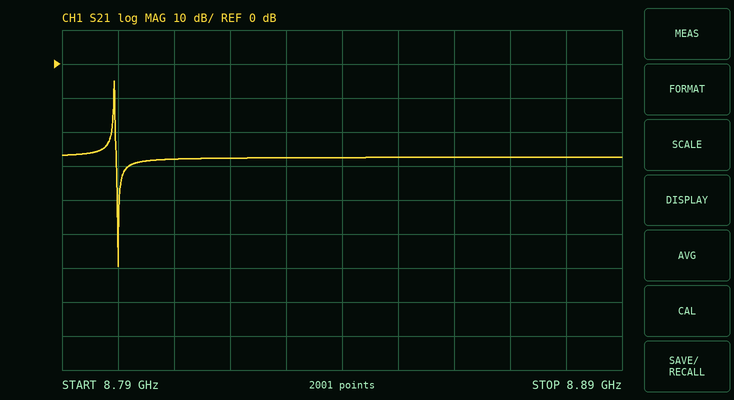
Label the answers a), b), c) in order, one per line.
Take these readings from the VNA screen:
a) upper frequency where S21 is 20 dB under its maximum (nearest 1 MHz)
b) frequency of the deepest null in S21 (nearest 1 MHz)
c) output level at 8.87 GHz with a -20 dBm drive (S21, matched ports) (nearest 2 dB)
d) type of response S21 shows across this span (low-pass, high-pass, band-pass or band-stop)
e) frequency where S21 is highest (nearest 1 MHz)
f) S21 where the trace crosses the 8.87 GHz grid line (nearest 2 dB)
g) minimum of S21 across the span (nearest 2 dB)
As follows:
a) 8.800 GHz
b) 8.800 GHz
c) -48 dBm
d) band-pass
e) 8.799 GHz
f) -28 dB
g) -60 dB
